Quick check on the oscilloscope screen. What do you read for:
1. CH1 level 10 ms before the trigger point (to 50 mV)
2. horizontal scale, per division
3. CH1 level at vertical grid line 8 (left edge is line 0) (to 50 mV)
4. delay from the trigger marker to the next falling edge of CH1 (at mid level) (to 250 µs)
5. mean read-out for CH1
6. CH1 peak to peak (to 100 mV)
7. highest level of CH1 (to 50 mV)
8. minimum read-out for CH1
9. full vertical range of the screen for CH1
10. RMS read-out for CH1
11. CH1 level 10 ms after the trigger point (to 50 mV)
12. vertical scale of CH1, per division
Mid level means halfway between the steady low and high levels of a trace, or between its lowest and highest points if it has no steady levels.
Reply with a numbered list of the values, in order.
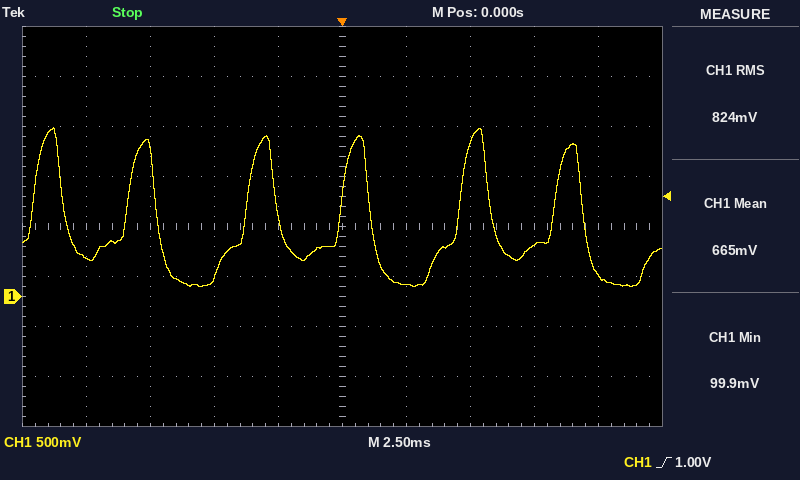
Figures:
1. 400 mV
2. 2.5 ms
3. 500 mV
4. 1.00 ms
5. 665 mV
6. 1.60 V
7. 1.70 V
8. 99.9 mV
9. 4 V
10. 824 mV
11. 200 mV
12. 500 mV
